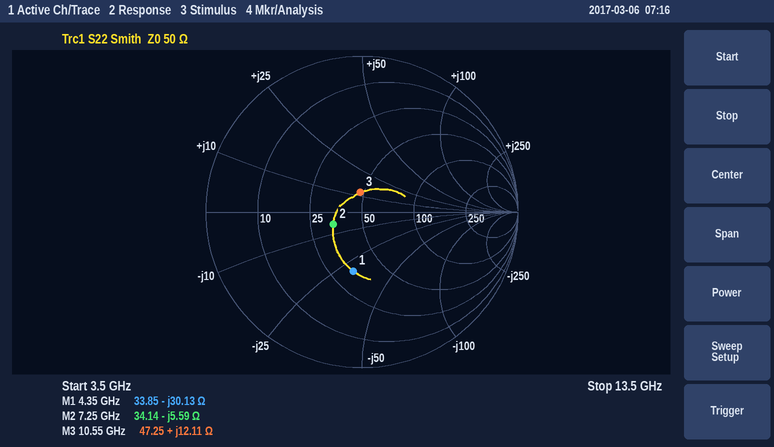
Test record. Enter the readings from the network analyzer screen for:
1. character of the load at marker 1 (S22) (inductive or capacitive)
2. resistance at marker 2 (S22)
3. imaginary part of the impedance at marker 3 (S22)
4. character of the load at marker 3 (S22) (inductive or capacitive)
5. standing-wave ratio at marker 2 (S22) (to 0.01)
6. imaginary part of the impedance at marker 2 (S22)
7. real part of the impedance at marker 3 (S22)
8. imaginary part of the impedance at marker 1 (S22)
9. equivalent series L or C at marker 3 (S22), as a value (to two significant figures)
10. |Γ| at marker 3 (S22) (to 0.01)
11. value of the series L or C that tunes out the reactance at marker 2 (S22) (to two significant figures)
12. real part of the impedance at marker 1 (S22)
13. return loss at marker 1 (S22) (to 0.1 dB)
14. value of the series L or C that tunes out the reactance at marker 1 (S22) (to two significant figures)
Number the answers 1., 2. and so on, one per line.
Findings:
1. capacitive
2. 34.14 Ω
3. +12.11 Ω
4. inductive
5. 1.50
6. -5.59 Ω
7. 47.25 Ω
8. -30.13 Ω
9. 180 pH
10. 0.13
11. 120 pH
12. 33.85 Ω
13. 8.3 dB
14. 1.1 nH
